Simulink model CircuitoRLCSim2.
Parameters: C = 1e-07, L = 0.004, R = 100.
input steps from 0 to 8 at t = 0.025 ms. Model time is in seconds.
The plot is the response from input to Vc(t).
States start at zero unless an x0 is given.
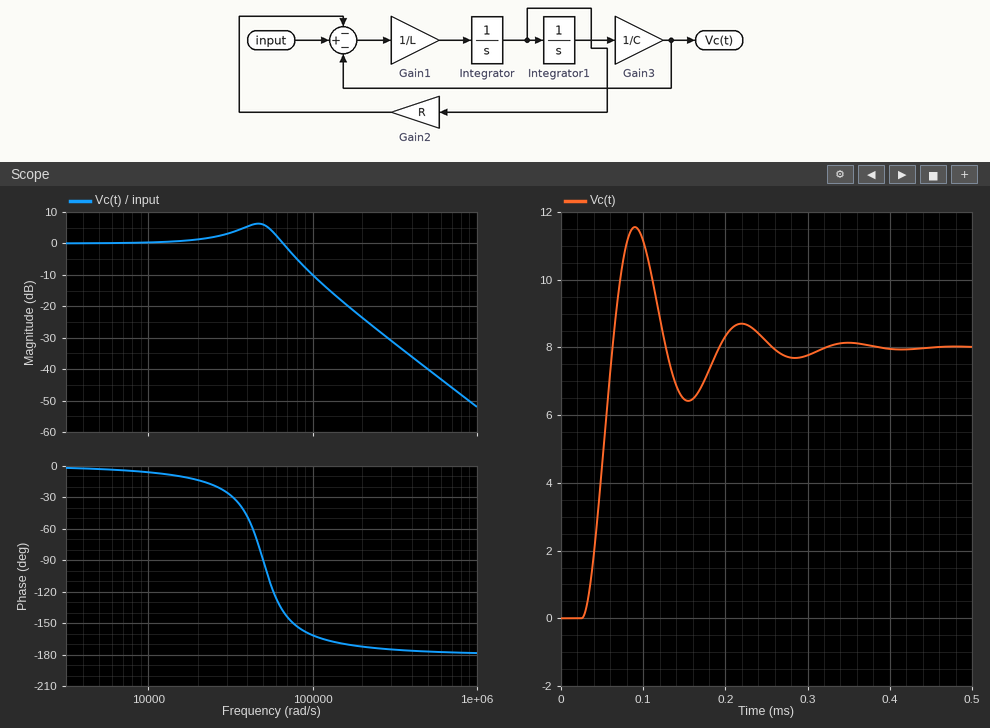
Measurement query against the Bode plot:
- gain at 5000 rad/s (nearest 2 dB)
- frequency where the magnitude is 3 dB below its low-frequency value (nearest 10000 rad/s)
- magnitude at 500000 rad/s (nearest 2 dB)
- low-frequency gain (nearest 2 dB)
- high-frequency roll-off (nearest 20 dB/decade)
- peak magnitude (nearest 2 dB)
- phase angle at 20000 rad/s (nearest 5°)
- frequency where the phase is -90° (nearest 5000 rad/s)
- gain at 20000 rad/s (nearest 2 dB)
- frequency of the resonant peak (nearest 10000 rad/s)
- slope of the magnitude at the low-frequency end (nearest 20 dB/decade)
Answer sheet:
0 dB
70000 rad/s
-40 dB
0 dB
-40 dB/decade
6 dB
-15°
50000 rad/s
2 dB
50000 rad/s
0 dB/decade
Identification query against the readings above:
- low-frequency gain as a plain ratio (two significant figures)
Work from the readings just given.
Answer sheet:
1.0
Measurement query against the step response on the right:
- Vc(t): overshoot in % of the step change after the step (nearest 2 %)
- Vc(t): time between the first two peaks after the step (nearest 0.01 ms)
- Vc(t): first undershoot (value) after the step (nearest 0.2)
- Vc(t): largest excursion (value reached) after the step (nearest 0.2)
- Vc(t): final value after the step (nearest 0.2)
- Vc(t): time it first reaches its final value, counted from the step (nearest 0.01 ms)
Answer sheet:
44 %
0.13 ms
6.4
11.6
8.0
0.04 ms
